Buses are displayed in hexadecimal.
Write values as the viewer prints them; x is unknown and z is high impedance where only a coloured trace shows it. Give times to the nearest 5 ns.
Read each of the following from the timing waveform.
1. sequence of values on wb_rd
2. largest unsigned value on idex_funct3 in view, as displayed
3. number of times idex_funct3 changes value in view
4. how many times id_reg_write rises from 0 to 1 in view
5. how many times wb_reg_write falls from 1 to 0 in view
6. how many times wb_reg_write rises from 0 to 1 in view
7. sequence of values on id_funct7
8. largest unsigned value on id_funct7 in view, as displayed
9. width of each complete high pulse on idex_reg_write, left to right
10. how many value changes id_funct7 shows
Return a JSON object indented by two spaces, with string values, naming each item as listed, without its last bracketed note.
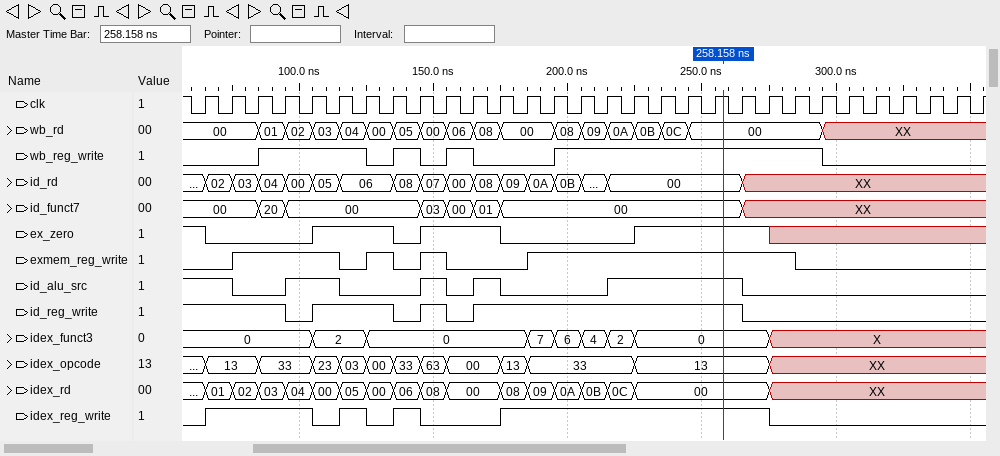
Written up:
{
  "sequence of values on wb_rd": "00, 01, 02, 03, 04, 00, 05, 00, 06, 08, 00, 08, 09, 0A, 0B, 0C, 00, XX",
  "largest unsigned value on idex_funct3 in view, as displayed": "7",
  "number of times idex_funct3 changes value in view": "8",
  "how many times id_reg_write rises from 0 to 1 in view": "3",
  "how many times wb_reg_write falls from 1 to 0 in view": "4",
  "how many times wb_reg_write rises from 0 to 1 in view": "4",
  "sequence of values on id_funct7": "00, 20, 00, 03, 00, 01, 00, XX",
  "largest unsigned value on id_funct7 in view, as displayed": "20",
  "width of each complete high pulse on idex_reg_write, left to right": "40 ns, 10 ns, 10 ns, 100 ns",
  "how many value changes id_funct7 shows": "7"
}
